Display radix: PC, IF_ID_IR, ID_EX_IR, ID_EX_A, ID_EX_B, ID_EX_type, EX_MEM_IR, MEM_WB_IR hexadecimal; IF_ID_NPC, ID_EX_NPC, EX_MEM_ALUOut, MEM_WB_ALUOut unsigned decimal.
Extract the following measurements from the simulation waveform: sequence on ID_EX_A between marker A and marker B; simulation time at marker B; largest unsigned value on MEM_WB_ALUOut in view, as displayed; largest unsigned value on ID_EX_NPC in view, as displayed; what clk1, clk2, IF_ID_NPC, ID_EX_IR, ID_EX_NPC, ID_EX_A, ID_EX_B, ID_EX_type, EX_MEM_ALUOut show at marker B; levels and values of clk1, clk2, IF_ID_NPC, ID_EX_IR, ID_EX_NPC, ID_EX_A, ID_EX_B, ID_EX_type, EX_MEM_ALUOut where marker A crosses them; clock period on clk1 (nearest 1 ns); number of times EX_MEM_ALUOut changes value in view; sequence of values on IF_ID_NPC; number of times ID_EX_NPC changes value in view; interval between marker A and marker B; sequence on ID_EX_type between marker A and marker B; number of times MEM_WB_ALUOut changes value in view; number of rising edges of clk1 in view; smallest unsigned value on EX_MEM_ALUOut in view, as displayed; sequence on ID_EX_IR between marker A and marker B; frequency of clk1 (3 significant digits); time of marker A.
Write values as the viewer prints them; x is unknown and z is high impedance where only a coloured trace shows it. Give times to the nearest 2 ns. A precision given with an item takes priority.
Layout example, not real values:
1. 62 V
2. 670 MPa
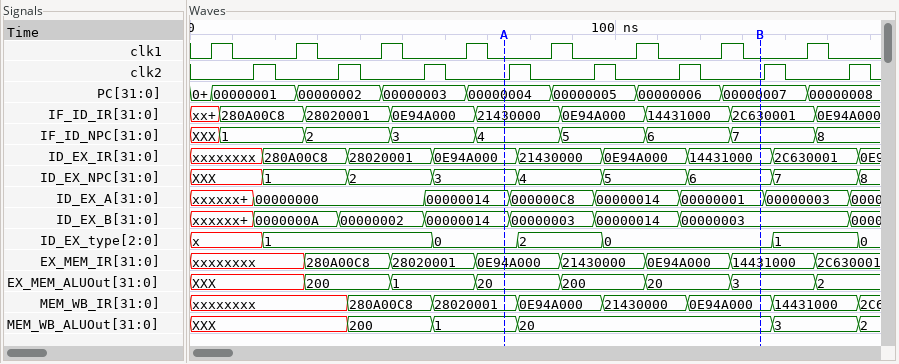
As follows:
1. 00000014, 000000C8, 00000014, 00000001
2. 134 ns
3. 200
4. 8
5. clk1=0, clk2=0, IF_ID_NPC=7, ID_EX_IR=14431000, ID_EX_NPC=6, ID_EX_A=00000001, ID_EX_B=00000003, ID_EX_type=0, EX_MEM_ALUOut=3
6. clk1=0, clk2=0, IF_ID_NPC=4, ID_EX_IR=0E94A000, ID_EX_NPC=3, ID_EX_A=00000014, ID_EX_B=00000014, ID_EX_type=0, EX_MEM_ALUOut=20
7. 20 ns
8. 7
9. XXX, 1, 2, 3, 4, 5, 6, 7, 8
10. 8
11. 60 ns
12. 0, 2, 0
13. 5
14. 8
15. 1
16. 0E94A000, 21430000, 0E94A000, 14431000
17. 50.0 MHz
18. 74 ns
